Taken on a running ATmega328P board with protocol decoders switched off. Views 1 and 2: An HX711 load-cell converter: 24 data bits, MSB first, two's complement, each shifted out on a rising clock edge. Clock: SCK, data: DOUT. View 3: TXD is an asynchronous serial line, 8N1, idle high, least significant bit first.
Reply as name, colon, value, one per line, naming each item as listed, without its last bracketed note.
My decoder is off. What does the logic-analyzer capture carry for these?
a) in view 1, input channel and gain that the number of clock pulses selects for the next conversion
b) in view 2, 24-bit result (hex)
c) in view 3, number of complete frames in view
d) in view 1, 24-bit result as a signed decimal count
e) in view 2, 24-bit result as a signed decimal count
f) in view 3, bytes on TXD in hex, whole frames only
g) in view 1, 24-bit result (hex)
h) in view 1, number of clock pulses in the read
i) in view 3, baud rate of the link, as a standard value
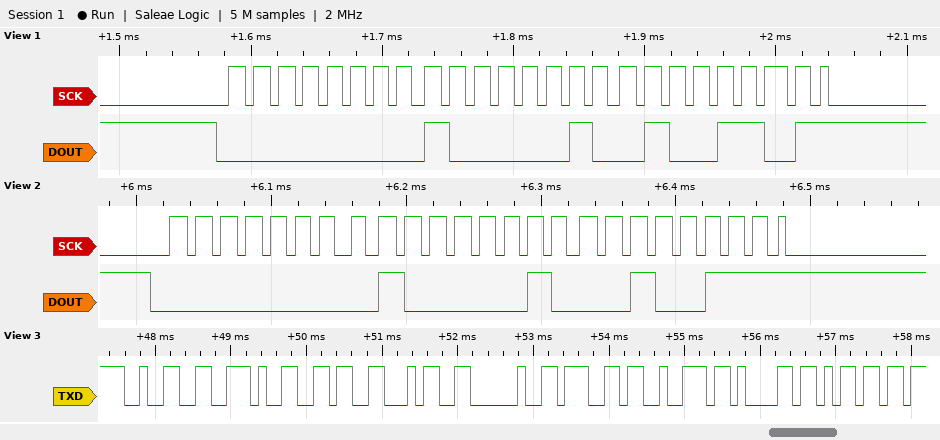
in view 1, input channel and gain that the number of clock pulses selects for the next conversion: channel A, gain 128
in view 2, 24-bit result: 0x008227
in view 3, number of complete frames in view: 9
in view 1, 24-bit result as a signed decimal count: 33357
in view 2, 24-bit result as a signed decimal count: 33319
in view 3, bytes on TXD in hex, whole frames only: 32 2E 36 34 20 67 72 61 6D
in view 1, 24-bit result: 0x00824D
in view 1, number of clock pulses in the read: 25
in view 3, baud rate of the link, as a standard value: 9600 baud
